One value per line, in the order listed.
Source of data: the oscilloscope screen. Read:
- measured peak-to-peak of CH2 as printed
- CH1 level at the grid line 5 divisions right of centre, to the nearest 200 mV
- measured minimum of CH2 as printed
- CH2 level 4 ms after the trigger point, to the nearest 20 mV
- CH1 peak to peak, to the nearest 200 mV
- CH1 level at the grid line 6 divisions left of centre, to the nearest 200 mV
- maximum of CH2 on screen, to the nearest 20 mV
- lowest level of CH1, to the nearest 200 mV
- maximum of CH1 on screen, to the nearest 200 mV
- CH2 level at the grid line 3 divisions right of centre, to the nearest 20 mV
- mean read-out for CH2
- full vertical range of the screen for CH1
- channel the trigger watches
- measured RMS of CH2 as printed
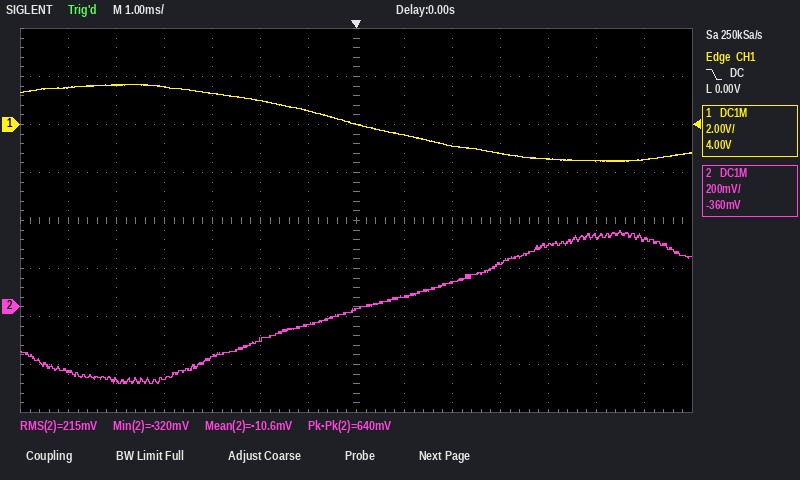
640 mV
-1.6 V
-320 mV
260 mV
3.2 V
1.6 V
320 mV
-1.6 V
1.6 V
180 mV
-10.6 mV
16 V
CH1
215 mV
